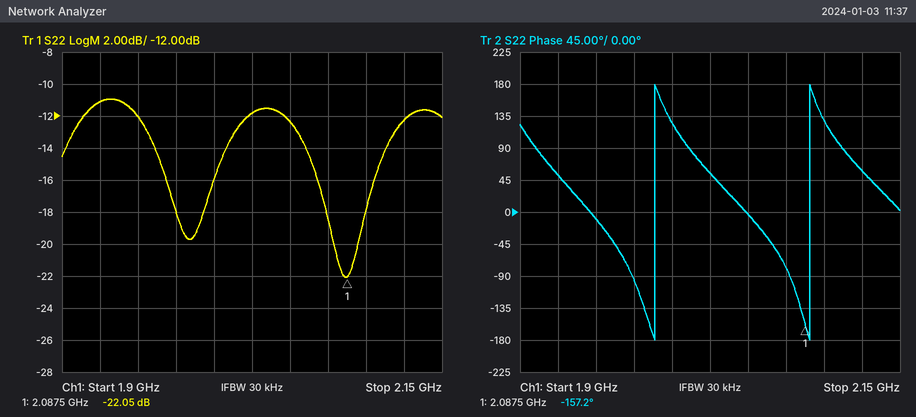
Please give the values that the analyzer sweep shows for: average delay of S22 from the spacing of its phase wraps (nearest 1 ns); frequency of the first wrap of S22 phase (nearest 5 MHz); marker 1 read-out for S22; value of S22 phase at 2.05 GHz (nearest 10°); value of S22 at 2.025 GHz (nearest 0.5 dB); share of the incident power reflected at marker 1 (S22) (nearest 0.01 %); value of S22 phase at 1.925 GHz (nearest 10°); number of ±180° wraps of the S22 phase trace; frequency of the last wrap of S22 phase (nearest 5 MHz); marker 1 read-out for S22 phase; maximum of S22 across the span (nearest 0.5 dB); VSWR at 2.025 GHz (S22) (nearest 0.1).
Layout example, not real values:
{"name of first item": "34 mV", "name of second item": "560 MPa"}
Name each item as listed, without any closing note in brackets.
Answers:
{"average delay of S22 from the spacing of its phase wraps": "10 ns", "frequency of the first wrap of S22 phase": "1.990 GHz", "marker 1 read-out for S22": "-22.05 dB", "value of S22 phase at 2.05 GHz": "0°", "value of S22 at 2.025 GHz": "-12.0 dB", "share of the incident power reflected at marker 1 (S22)": "0.62 %", "value of S22 phase at 1.925 GHz": "50°", "number of ±180° wraps of the S22 phase trace": "2", "frequency of the last wrap of S22 phase": "2.090 GHz", "marker 1 read-out for S22 phase": "-157.2°", "maximum of S22 across the span": "-11.0 dB", "VSWR at 2.025 GHz (S22)": "1.7"}
